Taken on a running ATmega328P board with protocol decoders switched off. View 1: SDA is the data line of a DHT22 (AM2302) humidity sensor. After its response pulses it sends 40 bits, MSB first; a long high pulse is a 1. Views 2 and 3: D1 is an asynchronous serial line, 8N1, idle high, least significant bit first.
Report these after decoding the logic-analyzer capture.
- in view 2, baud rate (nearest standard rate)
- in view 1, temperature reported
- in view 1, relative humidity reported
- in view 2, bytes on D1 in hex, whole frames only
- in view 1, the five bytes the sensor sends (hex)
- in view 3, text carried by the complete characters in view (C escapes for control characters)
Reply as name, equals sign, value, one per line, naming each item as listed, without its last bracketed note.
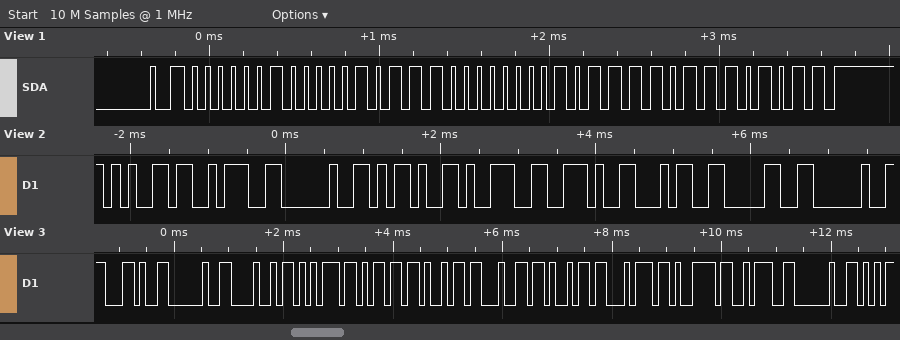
in view 2, baud rate = 9600 baud
in view 1, temperature reported = -9.4 °C
in view 1, relative humidity reported = 52.3 %
in view 2, bytes on D1 in hex, whole frames only = 65 3A 20 2D 39 2E 34 30 20
in view 1, the five bytes the sensor sends = 02 0B 80 5E EB
in view 3, text carried by the complete characters in view = ", Humidity: "
